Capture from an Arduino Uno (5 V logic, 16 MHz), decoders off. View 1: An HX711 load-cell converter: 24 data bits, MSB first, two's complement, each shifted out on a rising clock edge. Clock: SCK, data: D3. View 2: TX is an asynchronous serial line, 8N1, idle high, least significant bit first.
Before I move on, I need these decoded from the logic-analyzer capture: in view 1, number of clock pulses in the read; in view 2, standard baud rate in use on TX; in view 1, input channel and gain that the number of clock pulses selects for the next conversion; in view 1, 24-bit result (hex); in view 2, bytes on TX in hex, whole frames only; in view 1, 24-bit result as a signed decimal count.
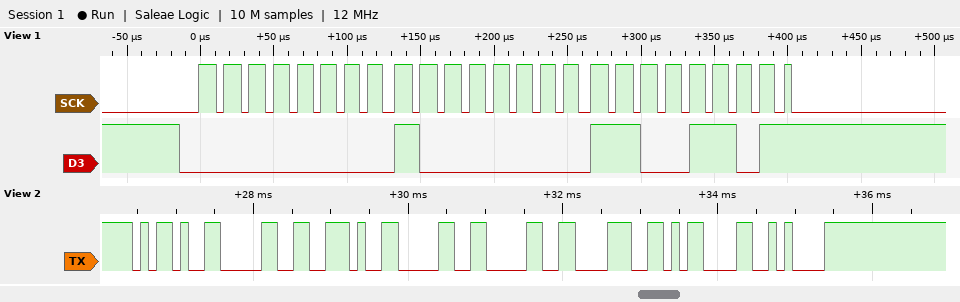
25
9600 baud
channel A, gain 128
0x0080CD
0x2D 0x30 0x2E 0x30 0x30 0x38 0x0D 0x0A
32973
